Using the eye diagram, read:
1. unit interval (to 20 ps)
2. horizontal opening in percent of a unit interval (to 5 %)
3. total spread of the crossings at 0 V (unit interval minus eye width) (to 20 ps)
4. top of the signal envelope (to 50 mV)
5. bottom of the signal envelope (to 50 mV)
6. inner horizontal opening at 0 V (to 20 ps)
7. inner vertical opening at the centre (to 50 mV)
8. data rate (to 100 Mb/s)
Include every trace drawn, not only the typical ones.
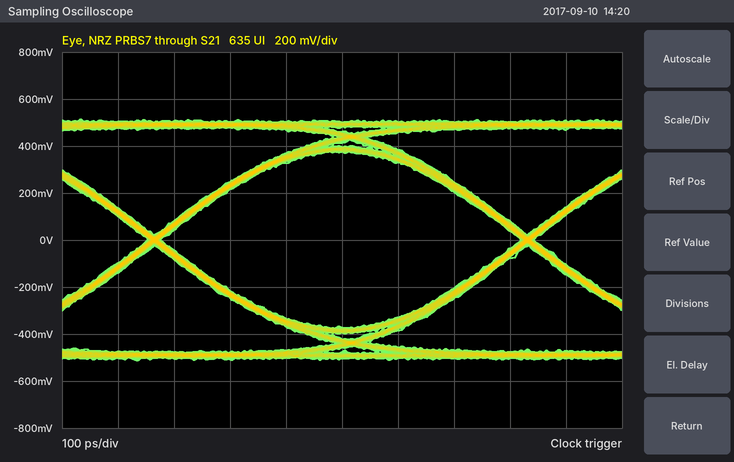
660 ps
95 %
20 ps
500 mV
-500 mV
640 ps
750 mV
1.5 Gb/s
